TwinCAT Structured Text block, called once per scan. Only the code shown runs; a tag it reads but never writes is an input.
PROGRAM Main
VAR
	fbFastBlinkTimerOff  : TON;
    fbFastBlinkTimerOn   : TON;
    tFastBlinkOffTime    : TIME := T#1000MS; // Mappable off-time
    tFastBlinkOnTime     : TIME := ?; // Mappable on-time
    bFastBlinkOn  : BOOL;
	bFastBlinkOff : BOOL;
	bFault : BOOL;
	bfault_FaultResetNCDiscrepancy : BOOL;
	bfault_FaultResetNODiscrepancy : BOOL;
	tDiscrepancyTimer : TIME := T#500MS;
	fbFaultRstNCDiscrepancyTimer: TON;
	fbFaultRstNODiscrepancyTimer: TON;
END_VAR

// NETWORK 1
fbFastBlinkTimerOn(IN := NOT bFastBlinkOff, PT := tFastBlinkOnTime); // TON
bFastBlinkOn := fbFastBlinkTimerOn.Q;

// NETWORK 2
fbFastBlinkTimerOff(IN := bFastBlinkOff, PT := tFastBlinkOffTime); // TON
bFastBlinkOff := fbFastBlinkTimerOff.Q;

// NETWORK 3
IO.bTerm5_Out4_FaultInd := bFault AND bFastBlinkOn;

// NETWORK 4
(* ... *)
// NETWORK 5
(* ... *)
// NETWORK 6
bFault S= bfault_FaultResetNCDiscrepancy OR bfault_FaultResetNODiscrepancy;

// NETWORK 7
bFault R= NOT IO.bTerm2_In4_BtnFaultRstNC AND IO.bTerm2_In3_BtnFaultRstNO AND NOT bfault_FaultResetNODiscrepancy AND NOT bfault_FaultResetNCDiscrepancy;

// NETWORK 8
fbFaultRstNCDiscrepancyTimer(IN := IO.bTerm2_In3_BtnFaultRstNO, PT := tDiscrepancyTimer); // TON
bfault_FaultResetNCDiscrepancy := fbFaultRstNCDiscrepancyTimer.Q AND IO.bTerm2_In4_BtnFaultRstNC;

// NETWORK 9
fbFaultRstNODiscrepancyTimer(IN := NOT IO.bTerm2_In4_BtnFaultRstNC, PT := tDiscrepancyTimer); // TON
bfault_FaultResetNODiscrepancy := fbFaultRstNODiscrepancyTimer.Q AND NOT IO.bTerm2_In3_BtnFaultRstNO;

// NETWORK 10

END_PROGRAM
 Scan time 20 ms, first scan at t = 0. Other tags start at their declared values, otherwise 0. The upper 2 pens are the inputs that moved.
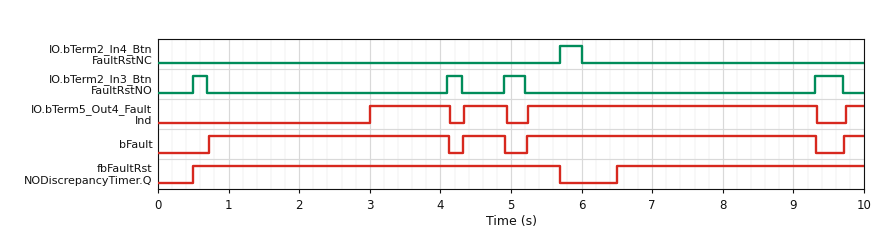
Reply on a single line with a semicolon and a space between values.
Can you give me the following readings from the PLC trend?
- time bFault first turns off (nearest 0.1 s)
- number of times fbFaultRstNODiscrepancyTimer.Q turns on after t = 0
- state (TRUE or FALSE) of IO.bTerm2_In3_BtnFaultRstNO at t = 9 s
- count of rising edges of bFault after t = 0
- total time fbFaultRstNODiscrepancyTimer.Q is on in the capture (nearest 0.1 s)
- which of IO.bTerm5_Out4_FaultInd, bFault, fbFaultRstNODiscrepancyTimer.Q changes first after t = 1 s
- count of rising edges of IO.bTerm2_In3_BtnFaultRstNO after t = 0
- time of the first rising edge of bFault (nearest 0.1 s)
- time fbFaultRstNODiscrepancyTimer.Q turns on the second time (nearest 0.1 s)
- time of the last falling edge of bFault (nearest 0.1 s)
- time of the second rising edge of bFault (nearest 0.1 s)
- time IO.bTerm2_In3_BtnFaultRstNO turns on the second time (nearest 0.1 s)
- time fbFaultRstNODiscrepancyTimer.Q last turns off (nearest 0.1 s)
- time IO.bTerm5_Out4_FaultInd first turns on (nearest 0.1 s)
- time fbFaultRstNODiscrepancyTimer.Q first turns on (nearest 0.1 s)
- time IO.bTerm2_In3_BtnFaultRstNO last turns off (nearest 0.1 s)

4.1 s; 2; FALSE; 4; 8.7 s; IO.bTerm5_Out4_FaultInd; 4; 0.7 s; 6.5 s; 9.3 s; 4.3 s; 4.1 s; 5.7 s; 3.0 s; 0.5 s; 9.7 s
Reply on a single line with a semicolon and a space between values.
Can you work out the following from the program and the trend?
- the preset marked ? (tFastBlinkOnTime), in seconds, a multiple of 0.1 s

3.0 s
